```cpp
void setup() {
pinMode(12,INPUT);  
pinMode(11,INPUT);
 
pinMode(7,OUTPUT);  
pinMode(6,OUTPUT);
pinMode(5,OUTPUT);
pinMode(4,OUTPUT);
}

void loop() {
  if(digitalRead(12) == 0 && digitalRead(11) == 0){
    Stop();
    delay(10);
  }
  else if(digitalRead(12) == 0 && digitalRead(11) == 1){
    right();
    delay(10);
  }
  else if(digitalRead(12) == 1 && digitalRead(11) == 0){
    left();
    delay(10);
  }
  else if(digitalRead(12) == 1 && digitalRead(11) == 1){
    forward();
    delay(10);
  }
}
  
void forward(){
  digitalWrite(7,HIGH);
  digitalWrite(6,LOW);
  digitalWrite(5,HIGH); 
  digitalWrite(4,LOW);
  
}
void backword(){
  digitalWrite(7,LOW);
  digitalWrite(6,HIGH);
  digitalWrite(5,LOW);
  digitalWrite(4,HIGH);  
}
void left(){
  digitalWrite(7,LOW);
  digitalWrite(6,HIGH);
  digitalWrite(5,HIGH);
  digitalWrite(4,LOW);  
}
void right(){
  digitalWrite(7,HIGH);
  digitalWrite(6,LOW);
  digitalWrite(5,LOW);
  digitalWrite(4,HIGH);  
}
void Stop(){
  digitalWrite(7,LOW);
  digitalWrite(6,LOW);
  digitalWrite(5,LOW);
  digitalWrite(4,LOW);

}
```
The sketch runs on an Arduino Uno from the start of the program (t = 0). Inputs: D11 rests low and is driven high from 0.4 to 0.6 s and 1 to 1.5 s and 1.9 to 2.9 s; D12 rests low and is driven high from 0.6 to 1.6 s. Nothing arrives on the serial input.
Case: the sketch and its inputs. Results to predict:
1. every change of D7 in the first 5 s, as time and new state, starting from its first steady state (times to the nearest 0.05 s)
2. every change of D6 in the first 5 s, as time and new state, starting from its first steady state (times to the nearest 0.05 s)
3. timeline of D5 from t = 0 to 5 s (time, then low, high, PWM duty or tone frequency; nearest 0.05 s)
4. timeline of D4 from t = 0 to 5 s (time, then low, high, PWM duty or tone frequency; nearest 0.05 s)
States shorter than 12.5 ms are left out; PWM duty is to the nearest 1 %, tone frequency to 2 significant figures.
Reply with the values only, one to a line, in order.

0 s low; 0.4 s high; 0.6 s low; 1 s high; 1.5 s low; 1.9 s high; 2.9 s low
0 s low; 0.6 s high; 1 s low; 1.5 s high; 1.6 s low
0 s low; 0.6 s high; 1.6 s low
0 s low; 0.4 s high; 0.6 s low; 1.9 s high; 2.9 s low
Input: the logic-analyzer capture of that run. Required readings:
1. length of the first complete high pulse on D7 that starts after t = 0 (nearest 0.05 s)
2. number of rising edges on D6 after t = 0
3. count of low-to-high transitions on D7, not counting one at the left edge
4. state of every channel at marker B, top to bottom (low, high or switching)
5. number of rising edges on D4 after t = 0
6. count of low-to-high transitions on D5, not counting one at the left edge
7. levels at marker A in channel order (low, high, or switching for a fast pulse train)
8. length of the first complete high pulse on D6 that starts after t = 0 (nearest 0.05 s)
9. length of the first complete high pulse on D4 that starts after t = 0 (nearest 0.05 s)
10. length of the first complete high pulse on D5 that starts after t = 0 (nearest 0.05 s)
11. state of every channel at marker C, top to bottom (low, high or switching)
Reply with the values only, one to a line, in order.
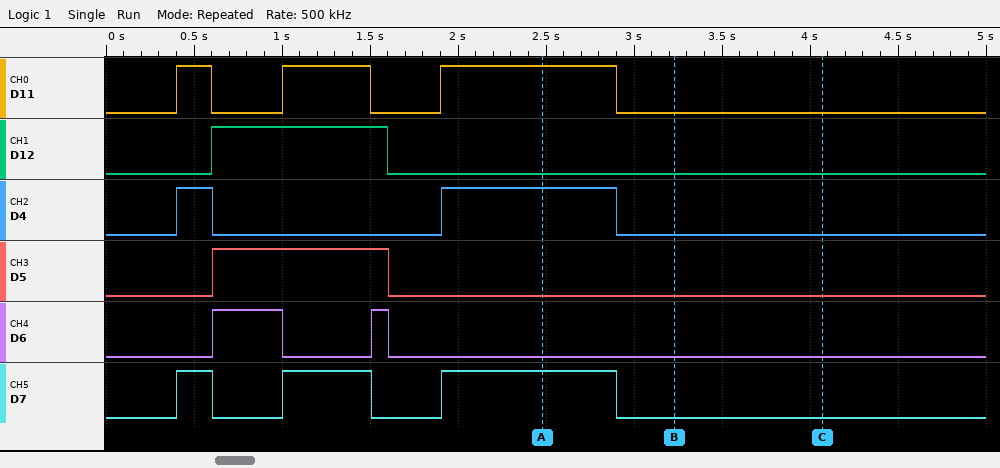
0.20 s
2
3
D11 low, D12 low, D4 low, D5 low, D6 low, D7 low
2
1
D11 high, D12 low, D4 high, D5 low, D6 low, D7 high
0.40 s
0.20 s
1.00 s
D11 low, D12 low, D4 low, D5 low, D6 low, D7 low
